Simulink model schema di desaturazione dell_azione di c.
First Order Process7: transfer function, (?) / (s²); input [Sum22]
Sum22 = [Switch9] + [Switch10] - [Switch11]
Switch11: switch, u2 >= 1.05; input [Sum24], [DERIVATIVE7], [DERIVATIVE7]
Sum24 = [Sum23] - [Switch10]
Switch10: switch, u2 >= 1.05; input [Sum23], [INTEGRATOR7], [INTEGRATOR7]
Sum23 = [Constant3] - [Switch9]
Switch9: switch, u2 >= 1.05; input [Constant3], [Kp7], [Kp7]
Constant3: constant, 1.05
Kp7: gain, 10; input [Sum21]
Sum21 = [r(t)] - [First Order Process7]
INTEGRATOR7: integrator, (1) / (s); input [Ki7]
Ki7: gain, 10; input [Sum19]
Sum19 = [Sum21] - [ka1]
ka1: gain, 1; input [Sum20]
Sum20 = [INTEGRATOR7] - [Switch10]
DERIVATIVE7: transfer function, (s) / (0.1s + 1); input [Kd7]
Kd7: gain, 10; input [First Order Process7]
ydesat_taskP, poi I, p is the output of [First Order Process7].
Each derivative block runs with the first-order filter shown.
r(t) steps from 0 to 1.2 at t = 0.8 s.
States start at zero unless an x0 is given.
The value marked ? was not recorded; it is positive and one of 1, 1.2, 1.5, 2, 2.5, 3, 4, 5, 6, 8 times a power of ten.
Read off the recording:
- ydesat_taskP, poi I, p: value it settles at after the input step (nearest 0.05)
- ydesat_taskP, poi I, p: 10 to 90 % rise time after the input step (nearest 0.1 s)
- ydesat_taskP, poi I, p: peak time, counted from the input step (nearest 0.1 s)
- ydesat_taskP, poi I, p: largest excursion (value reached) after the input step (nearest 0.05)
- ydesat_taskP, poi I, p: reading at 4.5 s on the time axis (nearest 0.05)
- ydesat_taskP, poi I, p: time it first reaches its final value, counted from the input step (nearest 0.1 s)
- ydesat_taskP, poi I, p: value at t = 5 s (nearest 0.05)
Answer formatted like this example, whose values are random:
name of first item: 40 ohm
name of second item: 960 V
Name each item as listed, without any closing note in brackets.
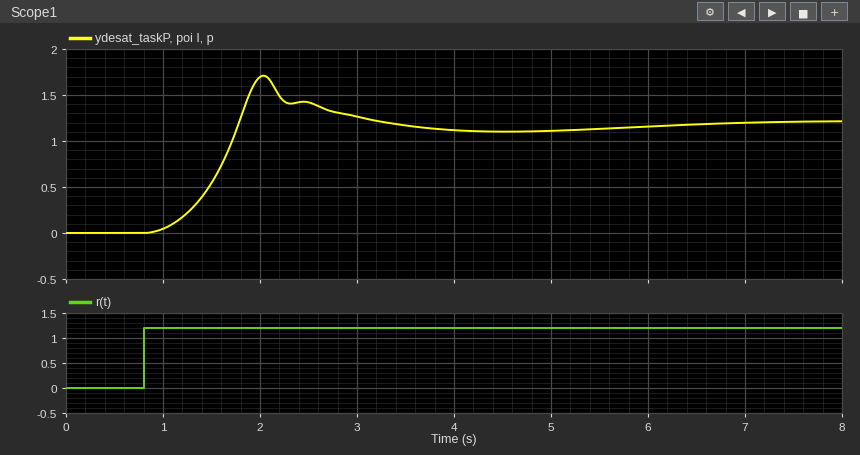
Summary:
ydesat_taskP, poi I, p: value it settles at after the input step: 1.20
ydesat_taskP, poi I, p: 10 to 90 % rise time after the input step: 0.6 s
ydesat_taskP, poi I, p: peak time, counted from the input step: 1.2 s
ydesat_taskP, poi I, p: largest excursion (value reached) after the input step: 1.70
ydesat_taskP, poi I, p: reading at 4.5 s on the time axis: 1.10
ydesat_taskP, poi I, p: time it first reaches its final value, counted from the input step: 1.0 s
ydesat_taskP, poi I, p: value at t = 5 s: 1.10
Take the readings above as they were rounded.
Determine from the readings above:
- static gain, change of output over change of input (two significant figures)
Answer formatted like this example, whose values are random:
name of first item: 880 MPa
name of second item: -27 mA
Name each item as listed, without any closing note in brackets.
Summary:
static gain, change of output over change of input: 1.0
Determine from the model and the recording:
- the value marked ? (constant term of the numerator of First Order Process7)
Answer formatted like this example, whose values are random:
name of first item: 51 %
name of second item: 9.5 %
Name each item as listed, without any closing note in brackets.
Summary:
the value marked ?: 2
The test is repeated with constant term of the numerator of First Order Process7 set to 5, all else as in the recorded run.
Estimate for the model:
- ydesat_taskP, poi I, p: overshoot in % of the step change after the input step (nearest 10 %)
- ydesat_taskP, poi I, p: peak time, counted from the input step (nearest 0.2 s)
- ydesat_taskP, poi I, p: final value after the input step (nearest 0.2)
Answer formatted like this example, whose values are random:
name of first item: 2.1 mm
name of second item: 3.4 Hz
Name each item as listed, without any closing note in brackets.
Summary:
ydesat_taskP, poi I, p: overshoot in % of the step change after the input step: 40 %
ydesat_taskP, poi I, p: peak time, counted from the input step: 0.8 s
ydesat_taskP, poi I, p: final value after the input step: 1.2
